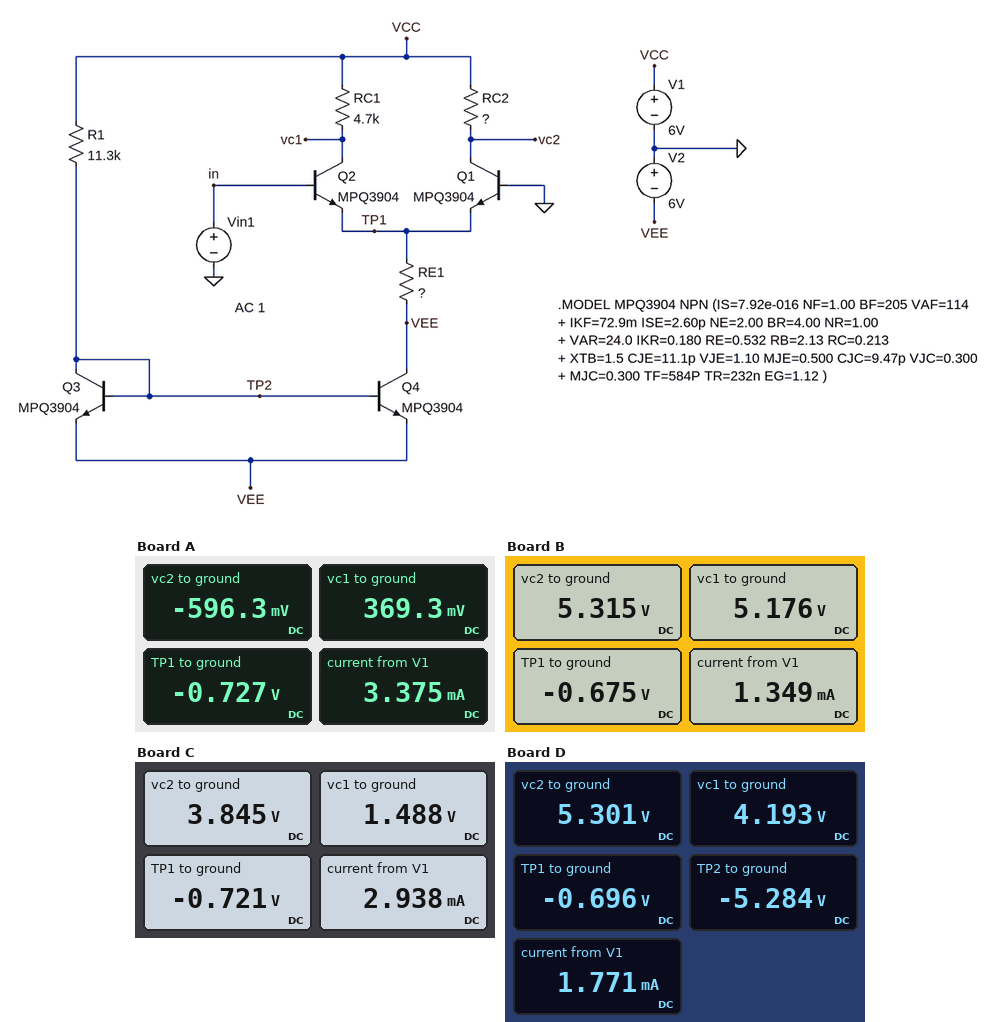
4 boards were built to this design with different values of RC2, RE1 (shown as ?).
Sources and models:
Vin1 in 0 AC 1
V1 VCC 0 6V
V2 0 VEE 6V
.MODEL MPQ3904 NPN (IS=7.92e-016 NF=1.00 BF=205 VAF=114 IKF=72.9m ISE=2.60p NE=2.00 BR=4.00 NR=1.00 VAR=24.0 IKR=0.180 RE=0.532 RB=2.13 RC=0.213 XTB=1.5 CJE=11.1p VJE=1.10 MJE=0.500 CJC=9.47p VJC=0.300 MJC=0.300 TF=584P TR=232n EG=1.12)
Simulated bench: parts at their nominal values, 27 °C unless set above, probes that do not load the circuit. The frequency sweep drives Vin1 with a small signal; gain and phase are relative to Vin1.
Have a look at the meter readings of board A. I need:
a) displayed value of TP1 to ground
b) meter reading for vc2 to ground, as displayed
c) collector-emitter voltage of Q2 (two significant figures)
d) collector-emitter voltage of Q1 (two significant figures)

-0.727 V
-596.3 mV
1.1 V
130 mV
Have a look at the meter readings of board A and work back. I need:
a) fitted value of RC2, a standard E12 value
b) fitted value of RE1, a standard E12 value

5.6 kΩ
2.2 kΩ
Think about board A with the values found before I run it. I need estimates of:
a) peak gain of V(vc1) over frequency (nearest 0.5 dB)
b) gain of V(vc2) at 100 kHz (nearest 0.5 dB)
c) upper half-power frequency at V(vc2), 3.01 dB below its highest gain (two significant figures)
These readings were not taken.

39.0 dB
34.0 dB
660 kHz
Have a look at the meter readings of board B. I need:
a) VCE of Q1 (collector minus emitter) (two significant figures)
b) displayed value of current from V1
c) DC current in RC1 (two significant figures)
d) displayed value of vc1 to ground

6.0 V
1.349 mA
180 µA
5.176 V
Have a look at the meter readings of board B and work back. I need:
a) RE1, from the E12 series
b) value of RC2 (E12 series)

15 kΩ
3.9 kΩ
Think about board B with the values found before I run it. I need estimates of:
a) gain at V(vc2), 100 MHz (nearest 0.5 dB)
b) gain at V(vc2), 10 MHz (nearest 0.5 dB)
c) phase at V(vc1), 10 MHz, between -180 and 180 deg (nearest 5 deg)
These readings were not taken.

2.5 dB
19.5 dB
125 deg
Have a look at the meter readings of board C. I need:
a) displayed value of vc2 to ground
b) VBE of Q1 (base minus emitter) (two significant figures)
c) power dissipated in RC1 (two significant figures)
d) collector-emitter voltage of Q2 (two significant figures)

3.845 V
720 mV
4.3 mW
2.2 V
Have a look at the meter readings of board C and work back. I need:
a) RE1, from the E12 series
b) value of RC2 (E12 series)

2.7 kΩ
2.2 kΩ
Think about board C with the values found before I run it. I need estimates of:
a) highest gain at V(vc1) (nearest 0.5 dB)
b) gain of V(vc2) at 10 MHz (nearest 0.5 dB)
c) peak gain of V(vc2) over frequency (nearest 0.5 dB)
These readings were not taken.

38.5 dB
30.0 dB
31.5 dB
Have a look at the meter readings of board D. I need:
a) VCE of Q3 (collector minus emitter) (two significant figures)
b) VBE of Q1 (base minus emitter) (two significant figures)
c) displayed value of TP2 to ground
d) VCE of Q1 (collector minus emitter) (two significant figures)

720 mV
700 mV
-5.284 V
6.0 V
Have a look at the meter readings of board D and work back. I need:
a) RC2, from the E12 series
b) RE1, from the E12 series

1.8 kΩ
6.8 kΩ
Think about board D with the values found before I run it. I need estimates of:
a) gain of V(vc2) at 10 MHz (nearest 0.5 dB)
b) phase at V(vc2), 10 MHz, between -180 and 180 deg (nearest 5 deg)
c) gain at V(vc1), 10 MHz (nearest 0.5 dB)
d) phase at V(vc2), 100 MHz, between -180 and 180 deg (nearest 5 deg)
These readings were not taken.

21.5 dB
-25 deg
26.5 dB
-80 deg
